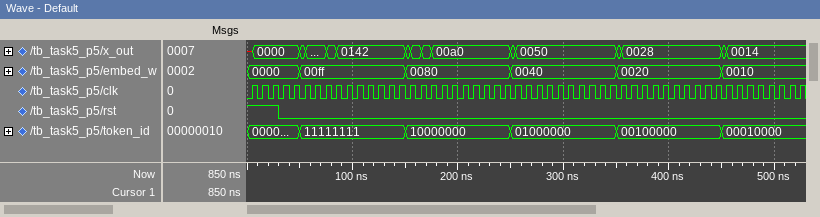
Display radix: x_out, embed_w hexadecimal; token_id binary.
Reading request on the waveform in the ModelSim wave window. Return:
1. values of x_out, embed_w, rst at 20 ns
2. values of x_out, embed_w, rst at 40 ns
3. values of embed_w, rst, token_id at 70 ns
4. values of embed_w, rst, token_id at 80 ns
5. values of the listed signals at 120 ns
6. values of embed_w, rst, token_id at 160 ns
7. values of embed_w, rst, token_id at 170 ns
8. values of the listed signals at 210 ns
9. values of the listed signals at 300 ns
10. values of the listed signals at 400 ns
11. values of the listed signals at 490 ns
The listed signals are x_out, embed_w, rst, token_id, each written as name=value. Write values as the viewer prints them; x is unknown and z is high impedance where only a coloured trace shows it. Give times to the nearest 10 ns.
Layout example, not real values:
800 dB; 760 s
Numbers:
x_out=0000, embed_w=0000, rst=1; x_out=0000, embed_w=0000, rst=0; embed_w=00ff, rst=0, token_id=11111111; embed_w=00ff, rst=0, token_id=11111111; x_out=0142, embed_w=00ff, rst=0, token_id=11111111; embed_w=0080, rst=0, token_id=10000000; embed_w=0080, rst=0, token_id=10000000; x_out=00a0, embed_w=0080, rst=0, token_id=10000000; x_out=0050, embed_w=0040, rst=0, token_id=01000000; x_out=0028, embed_w=0020, rst=0, token_id=00100000; x_out=0014, embed_w=0010, rst=0, token_id=00010000
